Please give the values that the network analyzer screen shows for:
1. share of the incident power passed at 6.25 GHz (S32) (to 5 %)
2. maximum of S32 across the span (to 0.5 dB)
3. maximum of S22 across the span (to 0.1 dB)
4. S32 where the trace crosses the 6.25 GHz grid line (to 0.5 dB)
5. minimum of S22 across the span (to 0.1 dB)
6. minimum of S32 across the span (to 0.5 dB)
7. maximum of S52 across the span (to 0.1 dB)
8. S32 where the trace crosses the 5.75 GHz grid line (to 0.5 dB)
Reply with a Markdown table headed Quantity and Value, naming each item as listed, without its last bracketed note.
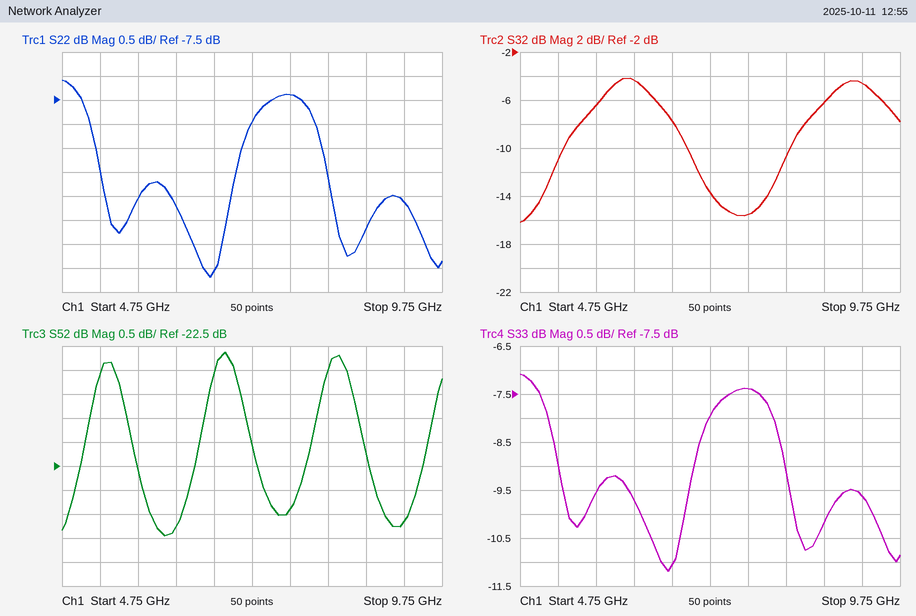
| Quantity | Value |
|---|---|
| share of the incident power passed at 6.25 GHz (S32) | 35 % |
| maximum of S32 across the span | -4.0 dB |
| maximum of S22 across the span | -7.1 dB |
| S32 where the trace crosses the 6.25 GHz grid line | -4.5 dB |
| minimum of S22 across the span | -11.2 dB |
| minimum of S32 across the span | -16.0 dB |
| maximum of S52 across the span | -20.1 dB |
| S32 where the trace crosses the 5.75 GHz grid line | -6.5 dB |
